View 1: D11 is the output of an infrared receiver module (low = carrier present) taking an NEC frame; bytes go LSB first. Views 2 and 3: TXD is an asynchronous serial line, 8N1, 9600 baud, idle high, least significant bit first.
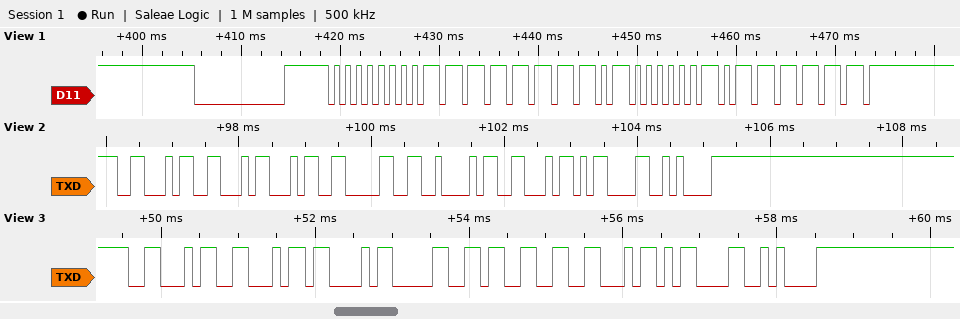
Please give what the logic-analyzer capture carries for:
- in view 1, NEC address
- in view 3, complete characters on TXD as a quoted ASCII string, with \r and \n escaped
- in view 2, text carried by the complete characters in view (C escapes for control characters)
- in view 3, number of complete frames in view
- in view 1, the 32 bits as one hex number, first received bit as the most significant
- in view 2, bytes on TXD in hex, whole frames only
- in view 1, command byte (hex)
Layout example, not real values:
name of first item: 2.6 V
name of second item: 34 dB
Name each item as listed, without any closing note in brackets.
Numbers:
in view 1, NEC address: 0x00
in view 3, complete characters on TXD as a quoted ASCII string, with \r and \n escaped: "FFC03F\r\n"
in view 2, text carried by the complete characters in view: "FF40BF\r\n"
in view 3, number of complete frames in view: 8
in view 1, the 32 bits as one hex number, first received bit as the most significant: 0x00FF40BF
in view 2, bytes on TXD in hex, whole frames only: 46 46 34 30 42 46 0D 0A
in view 1, command byte: 0x02
